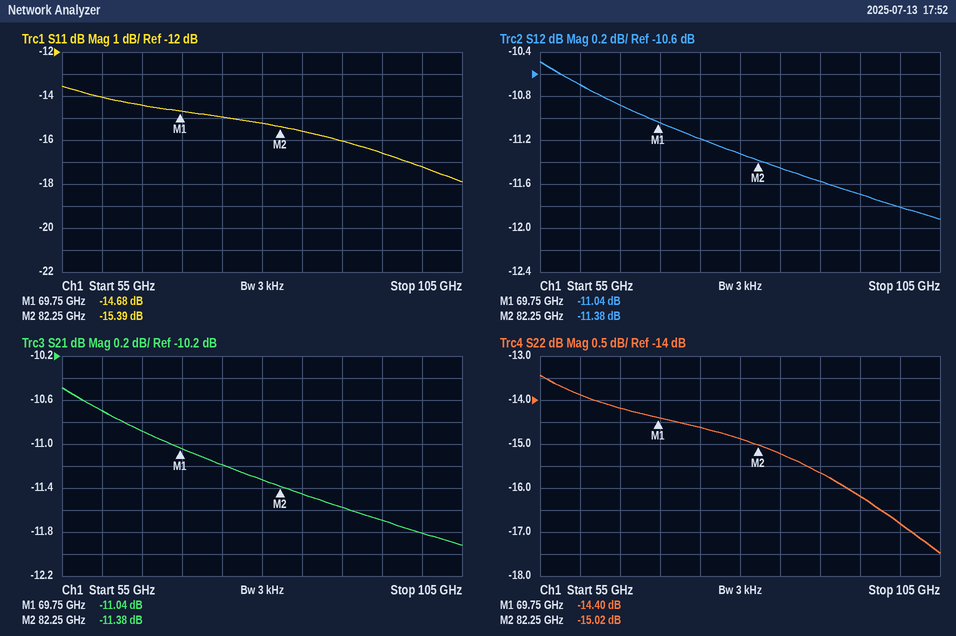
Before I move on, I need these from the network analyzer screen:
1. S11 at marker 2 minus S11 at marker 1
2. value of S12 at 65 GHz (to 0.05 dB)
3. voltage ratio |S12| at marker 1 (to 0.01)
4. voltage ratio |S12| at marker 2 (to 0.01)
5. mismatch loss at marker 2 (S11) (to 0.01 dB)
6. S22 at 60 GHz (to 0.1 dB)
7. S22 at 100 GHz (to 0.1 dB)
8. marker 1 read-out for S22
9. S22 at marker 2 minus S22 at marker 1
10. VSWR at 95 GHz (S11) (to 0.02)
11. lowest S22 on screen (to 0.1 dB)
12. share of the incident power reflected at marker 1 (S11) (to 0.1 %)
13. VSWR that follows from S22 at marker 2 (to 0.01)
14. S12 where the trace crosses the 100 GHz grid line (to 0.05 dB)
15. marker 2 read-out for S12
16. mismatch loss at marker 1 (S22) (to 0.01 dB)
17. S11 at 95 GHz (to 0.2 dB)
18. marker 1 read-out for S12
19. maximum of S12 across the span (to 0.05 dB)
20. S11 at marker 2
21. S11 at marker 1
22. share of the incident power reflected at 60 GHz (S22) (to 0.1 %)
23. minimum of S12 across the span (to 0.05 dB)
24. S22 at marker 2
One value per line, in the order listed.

-0.71 dB
-10.90 dB
0.28
0.27
0.13 dB
-13.9 dB
-16.8 dB
-14.40 dB
-0.62 dB
1.34
-17.5 dB
3.4 %
1.43
-11.80 dB
-11.38 dB
0.16 dB
-16.6 dB
-11.04 dB
-10.50 dB
-15.39 dB
-14.68 dB
4.1 %
-11.90 dB
-15.02 dB
